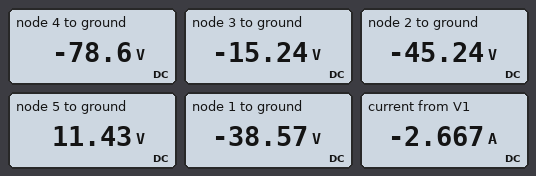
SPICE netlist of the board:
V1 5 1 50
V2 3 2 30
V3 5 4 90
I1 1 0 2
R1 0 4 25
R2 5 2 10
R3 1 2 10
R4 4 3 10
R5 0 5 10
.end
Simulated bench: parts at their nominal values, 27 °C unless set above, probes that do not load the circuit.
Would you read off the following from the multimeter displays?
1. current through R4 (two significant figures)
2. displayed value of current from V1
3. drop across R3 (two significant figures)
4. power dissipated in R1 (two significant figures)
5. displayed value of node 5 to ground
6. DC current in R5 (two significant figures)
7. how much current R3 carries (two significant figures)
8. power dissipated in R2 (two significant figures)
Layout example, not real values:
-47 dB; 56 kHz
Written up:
6.3 A; -2.667 A; 6.7 V; 250 W; 11.43 V; 1.1 A; 670 mA; 320 W
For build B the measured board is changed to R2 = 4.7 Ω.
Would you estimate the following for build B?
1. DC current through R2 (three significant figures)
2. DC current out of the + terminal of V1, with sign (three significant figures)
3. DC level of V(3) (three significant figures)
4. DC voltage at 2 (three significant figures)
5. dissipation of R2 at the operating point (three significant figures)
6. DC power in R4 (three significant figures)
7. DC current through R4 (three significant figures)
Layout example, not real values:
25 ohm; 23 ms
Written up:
8.76 A; -1.12 A; 243 mV; -29.8 V; 361 W; 621 W; 7.88 A
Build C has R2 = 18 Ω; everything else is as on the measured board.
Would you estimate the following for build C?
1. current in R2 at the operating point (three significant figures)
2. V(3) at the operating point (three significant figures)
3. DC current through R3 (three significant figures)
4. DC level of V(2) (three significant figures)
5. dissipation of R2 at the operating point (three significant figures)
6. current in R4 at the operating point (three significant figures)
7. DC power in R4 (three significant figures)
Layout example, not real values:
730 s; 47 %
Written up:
3.70 A; -25.1 V; 1.65 A; -55.1 V; 246 W; 5.35 A; 286 W
